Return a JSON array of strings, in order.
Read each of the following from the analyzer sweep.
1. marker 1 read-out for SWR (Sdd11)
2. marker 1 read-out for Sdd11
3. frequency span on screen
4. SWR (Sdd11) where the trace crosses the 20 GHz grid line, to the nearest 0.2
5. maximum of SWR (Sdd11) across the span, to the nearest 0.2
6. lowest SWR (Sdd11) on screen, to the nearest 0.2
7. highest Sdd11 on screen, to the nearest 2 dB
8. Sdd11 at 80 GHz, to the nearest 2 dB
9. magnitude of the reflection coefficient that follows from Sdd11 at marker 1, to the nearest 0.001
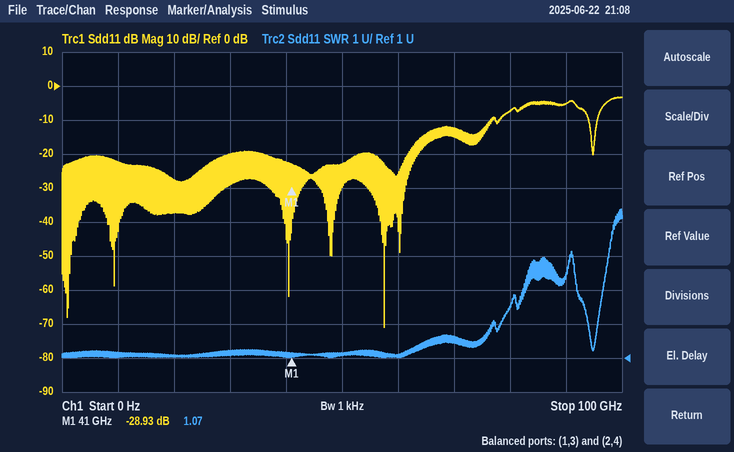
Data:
["1.07", "-28.93 dB", "100 GHz", "1.0", "5.4", "1.0", "-4 dB", "-8 dB", "0.036"]
